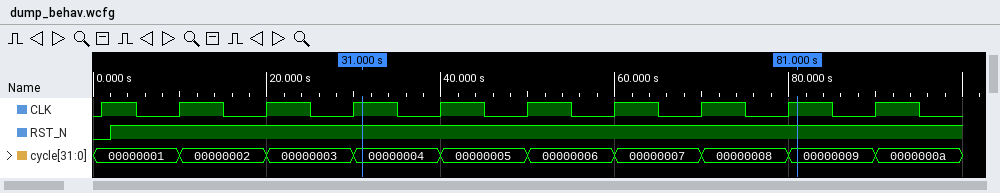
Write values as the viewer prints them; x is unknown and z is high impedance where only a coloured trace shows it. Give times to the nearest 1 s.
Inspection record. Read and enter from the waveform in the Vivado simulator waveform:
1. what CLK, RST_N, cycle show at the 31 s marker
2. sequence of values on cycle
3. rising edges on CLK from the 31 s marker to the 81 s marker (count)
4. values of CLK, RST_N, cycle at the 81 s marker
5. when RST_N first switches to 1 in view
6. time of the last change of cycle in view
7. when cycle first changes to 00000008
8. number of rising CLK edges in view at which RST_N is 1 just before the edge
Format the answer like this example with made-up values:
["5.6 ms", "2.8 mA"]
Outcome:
["CLK=1, RST_N=1, cycle=00000004", "00000001, 00000002, 00000003, 00000004, 00000005, 00000006, 00000007, 00000008, 00000009, 0000000a", "5", "CLK=1, RST_N=1, cycle=00000009", "2 s", "90 s", "70 s", "9"]
